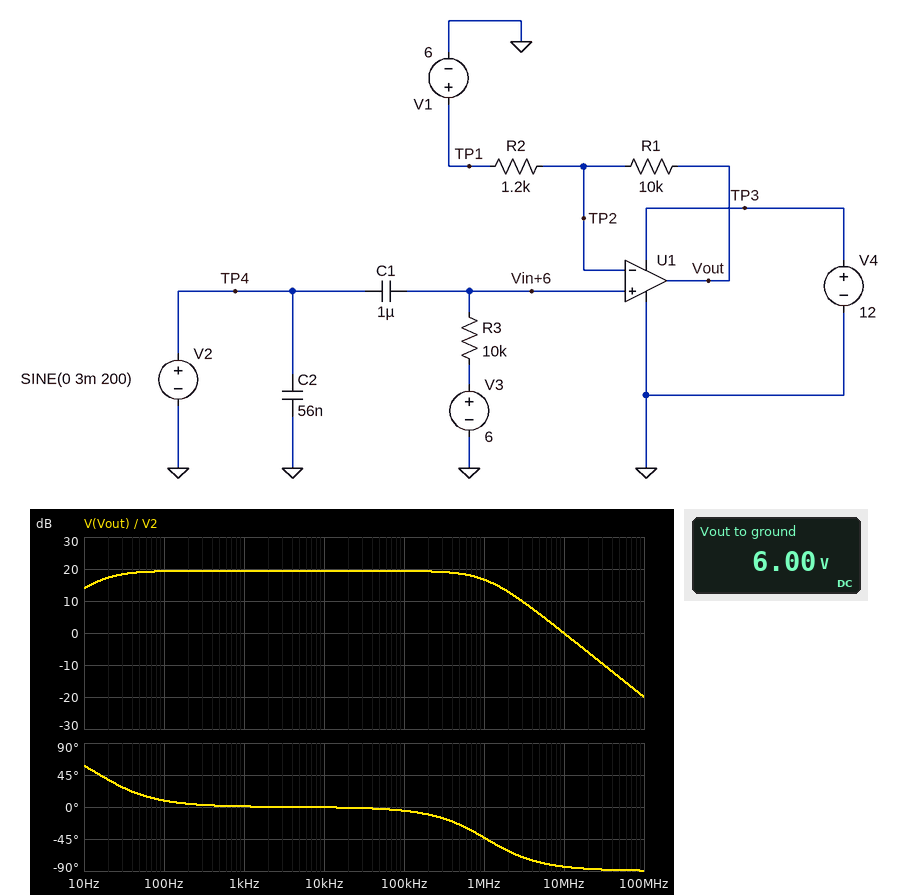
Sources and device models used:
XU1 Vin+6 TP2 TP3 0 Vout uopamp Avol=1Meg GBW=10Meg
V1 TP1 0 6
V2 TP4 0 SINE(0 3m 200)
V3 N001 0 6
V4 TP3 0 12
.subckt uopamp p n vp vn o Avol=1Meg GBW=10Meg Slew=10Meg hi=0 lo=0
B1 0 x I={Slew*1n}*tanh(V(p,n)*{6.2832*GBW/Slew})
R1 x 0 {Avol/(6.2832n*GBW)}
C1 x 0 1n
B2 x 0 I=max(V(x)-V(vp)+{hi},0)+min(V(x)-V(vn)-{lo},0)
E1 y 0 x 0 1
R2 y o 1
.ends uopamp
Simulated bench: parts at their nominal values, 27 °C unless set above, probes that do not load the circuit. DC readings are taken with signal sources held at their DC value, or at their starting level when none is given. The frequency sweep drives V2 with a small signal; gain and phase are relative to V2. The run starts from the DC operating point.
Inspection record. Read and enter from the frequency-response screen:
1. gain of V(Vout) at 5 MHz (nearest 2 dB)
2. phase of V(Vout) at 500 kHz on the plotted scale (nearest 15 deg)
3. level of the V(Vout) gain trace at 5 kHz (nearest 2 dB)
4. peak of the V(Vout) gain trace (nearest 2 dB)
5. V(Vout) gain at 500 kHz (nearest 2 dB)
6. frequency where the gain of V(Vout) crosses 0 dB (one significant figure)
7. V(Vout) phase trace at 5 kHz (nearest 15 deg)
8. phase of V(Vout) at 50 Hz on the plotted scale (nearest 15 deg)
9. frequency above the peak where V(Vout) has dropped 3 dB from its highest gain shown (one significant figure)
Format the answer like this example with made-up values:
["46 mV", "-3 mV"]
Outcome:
["6 dB", "-30 deg", "20 dB", "20 dB", "18 dB", "10 MHz", "0 deg", "15 deg", "1 MHz"]
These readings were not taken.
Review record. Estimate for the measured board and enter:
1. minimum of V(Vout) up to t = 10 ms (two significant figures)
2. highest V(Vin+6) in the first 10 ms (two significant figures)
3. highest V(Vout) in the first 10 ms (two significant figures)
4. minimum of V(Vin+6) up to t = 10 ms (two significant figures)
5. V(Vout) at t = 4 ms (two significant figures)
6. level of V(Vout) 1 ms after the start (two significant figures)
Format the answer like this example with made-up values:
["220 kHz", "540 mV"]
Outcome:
["6.0 V", "6.0 V", "6.0 V", "6.0 V", "6.0 V", "6.0 V"]
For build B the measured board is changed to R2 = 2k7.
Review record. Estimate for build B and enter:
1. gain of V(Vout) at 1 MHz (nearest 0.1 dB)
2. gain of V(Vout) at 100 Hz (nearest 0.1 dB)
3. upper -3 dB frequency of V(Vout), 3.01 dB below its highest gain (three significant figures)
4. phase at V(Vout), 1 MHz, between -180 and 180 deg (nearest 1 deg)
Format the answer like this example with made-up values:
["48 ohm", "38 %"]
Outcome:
["12.6 dB", "13.3 dB", "2.13 MHz", "-25 deg"]
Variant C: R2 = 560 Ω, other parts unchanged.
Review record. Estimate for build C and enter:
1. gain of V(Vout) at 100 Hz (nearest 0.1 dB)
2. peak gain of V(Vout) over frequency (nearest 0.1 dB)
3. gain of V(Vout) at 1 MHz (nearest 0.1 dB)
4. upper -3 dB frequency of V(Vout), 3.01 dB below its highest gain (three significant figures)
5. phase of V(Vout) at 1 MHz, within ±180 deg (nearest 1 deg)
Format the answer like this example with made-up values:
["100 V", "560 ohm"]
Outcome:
["25.4 dB", "25.5 dB", "18.9 dB", "530 kHz", "-62 deg"]
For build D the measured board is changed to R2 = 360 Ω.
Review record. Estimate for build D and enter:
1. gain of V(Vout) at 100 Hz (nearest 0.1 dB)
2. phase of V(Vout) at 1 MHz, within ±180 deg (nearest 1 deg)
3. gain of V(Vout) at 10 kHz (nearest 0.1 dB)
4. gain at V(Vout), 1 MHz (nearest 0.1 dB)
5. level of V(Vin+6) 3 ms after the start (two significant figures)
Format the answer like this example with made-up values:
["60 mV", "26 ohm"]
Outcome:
["29.1 dB", "-71 deg", "29.2 dB", "19.5 dB", "6.0 V"]
